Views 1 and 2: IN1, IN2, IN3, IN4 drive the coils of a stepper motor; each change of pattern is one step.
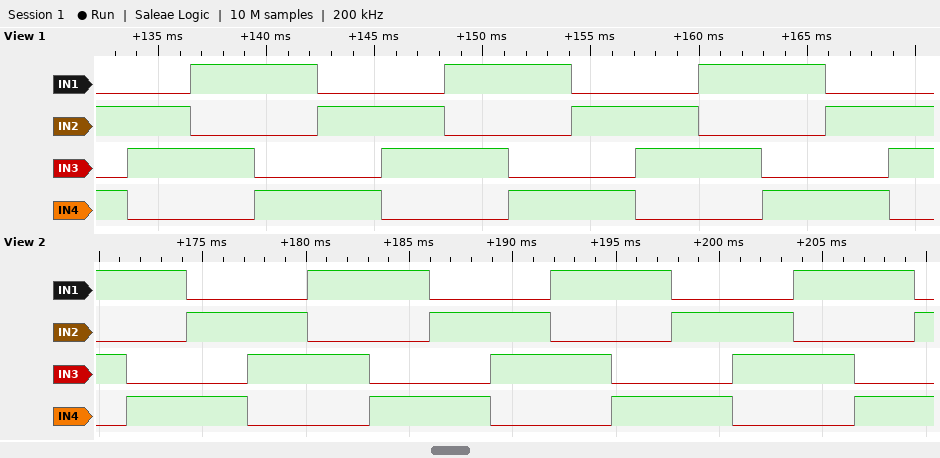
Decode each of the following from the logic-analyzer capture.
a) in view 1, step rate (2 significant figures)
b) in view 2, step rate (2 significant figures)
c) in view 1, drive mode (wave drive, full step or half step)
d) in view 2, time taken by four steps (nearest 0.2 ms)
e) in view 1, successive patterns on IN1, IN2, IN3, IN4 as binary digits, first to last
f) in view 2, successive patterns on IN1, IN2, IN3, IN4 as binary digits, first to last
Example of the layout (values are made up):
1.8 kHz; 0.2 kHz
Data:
340 steps/s; 340 steps/s; full step; 11.8 ms; 0101 0110 1010 1001 0101 0110 1010 1001 0101 0110 1010 1001 0101 0110; 1010 1001 0101 0110 1010 1001 0101 0110 1010 1001 0101 0110 1010 1001 0101
